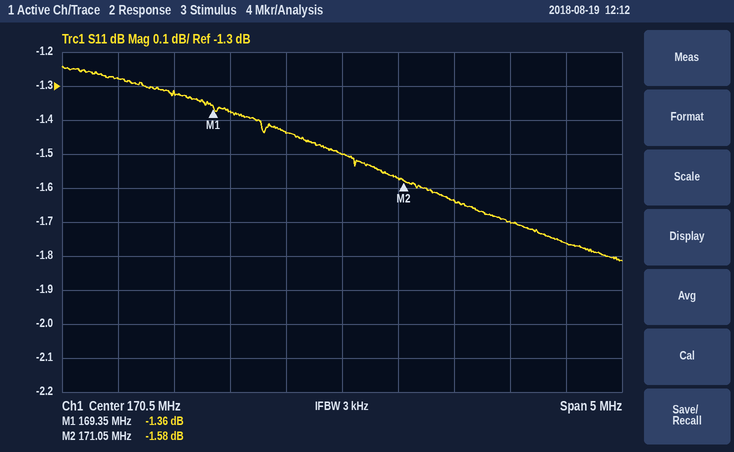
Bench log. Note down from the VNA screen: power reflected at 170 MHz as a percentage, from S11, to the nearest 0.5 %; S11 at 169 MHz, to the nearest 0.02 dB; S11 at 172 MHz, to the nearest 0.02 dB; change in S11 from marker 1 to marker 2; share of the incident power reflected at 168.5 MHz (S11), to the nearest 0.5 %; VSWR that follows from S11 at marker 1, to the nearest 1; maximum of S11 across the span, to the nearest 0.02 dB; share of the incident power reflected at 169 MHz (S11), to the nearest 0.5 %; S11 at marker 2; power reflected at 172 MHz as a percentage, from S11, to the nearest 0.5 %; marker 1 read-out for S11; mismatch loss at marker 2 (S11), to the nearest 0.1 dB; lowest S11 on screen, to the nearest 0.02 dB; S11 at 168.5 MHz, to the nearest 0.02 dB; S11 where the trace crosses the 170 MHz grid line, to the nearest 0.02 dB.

72.0 %
-1.32 dB
-1.70 dB
-0.22 dB
74.5 %
13
-1.24 dB
74.0 %
-1.58 dB
67.5 %
-1.36 dB
5.2 dB
-1.82 dB
-1.28 dB
-1.44 dB
